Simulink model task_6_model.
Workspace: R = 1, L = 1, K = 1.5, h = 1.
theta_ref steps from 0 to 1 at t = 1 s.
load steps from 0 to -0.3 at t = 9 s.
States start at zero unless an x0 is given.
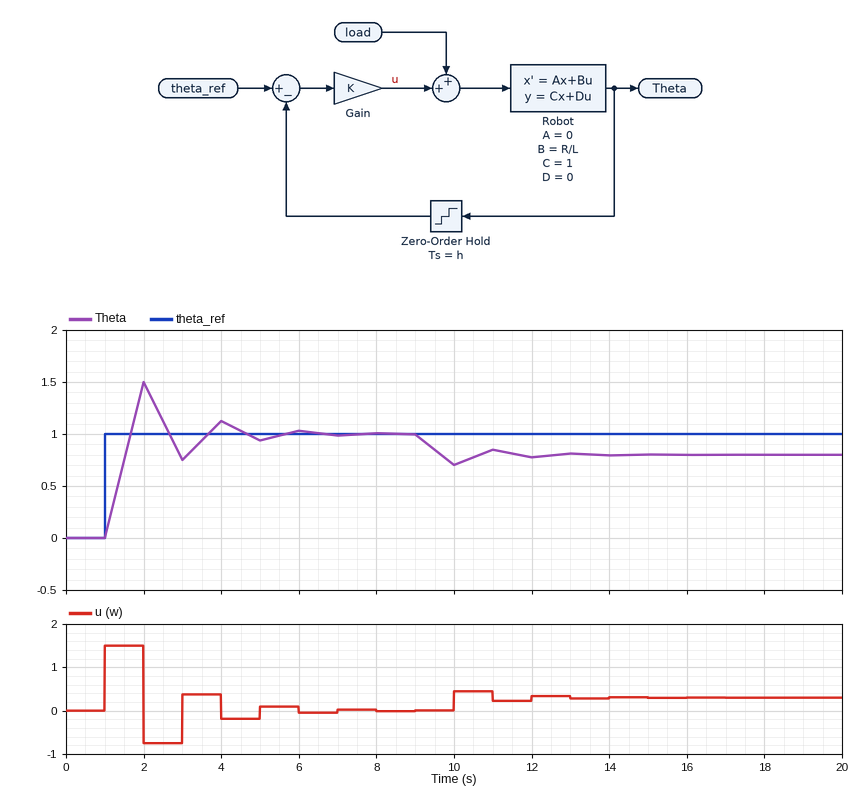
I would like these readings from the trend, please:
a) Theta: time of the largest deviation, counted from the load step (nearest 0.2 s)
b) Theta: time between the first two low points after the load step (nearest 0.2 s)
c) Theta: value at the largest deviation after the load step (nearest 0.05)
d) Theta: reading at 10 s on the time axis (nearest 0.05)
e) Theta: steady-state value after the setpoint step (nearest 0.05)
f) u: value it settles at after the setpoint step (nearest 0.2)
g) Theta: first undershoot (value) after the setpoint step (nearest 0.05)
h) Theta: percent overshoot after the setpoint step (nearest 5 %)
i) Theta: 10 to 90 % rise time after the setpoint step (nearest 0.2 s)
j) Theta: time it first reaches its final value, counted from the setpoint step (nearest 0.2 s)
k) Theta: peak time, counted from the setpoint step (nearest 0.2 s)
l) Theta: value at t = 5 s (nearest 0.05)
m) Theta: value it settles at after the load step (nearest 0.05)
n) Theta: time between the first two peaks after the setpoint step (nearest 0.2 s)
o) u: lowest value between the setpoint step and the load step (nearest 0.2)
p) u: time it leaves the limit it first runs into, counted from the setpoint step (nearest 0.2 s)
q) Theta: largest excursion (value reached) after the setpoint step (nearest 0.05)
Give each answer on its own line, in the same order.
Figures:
1.0 s
2.0 s
0.70
0.70
1.00
0.0
0.75
50 %
0.6 s
0.6 s
1.0 s
0.95
0.80
2.0 s
-0.8
1.0 s
1.50
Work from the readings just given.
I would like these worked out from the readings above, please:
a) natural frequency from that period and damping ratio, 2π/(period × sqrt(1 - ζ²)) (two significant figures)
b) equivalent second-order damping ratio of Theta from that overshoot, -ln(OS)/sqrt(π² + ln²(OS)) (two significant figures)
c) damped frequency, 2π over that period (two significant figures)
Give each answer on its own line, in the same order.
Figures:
3.2 rad/s
0.22
3.1 rad/s
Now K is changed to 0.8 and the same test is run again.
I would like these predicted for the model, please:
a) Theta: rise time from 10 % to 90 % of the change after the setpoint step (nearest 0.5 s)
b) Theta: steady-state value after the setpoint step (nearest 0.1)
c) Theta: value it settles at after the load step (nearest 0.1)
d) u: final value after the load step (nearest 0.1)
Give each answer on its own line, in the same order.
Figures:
1.5 s
1.0
0.6
0.3
